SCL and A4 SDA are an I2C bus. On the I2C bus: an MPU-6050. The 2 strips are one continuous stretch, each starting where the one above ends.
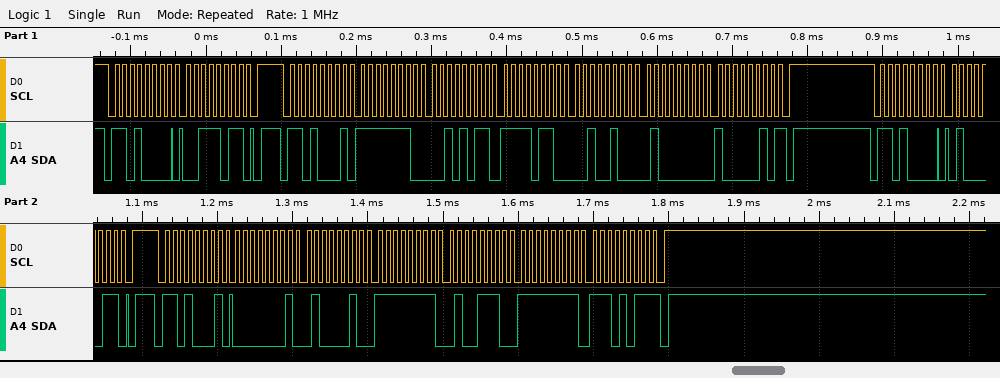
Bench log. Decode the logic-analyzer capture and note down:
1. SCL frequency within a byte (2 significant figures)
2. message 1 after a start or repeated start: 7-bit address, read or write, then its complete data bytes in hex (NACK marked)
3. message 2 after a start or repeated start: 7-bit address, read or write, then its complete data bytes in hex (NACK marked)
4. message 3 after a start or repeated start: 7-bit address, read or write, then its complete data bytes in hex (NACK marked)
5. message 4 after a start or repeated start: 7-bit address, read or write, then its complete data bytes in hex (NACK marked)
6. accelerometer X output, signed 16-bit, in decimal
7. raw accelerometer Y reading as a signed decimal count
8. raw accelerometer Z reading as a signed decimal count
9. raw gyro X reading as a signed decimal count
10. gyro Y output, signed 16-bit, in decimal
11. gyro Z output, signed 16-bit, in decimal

100 kHz
0x68 write: 3B
0x68 read: FE 2B F6 24 40 82 NACK
0x68 write: 43
0x68 read: 01 42 FF 4E FF EB NACK
-469
-2524
16514
322
-178
-21
